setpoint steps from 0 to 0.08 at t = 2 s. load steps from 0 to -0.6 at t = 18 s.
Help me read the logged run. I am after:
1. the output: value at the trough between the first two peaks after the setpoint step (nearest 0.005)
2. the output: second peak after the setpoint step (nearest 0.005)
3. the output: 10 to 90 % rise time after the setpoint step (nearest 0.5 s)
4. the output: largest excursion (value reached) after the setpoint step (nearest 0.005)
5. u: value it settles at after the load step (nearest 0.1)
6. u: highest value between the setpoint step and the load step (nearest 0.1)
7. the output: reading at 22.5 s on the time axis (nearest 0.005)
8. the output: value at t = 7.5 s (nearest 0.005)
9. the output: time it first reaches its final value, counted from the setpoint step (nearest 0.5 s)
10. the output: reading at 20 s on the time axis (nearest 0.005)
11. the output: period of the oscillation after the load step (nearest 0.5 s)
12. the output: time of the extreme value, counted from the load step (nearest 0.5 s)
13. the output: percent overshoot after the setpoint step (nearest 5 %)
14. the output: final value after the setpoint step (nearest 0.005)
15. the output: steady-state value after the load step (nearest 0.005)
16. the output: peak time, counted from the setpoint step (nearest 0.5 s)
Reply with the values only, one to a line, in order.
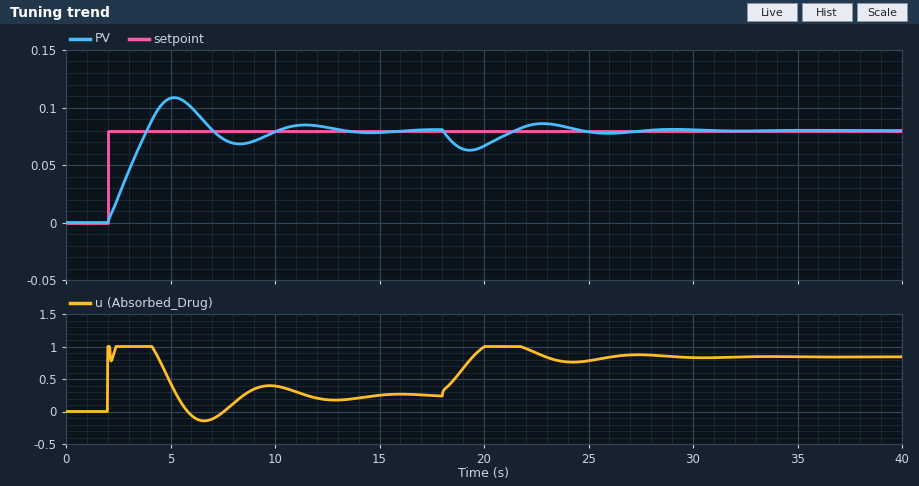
0.070
0.085
1.5 s
0.110
0.8
1.0
0.085
0.075
2.0 s
0.065
6.5 s
1.5 s
35 %
0.080
0.080
3.0 s
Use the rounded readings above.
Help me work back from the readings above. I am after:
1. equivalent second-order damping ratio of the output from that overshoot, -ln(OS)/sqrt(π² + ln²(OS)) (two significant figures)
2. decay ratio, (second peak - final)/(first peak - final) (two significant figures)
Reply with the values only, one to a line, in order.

0.32
0.17
